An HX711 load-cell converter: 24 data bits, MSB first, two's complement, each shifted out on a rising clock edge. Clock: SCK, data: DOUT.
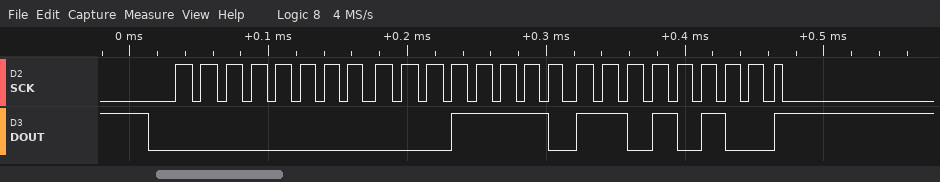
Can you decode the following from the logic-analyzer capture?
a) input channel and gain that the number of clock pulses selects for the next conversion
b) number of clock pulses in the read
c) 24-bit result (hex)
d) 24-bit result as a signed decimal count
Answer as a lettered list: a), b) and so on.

a) channel A, gain 128
b) 25
c) 0x001ED4
d) 7892
